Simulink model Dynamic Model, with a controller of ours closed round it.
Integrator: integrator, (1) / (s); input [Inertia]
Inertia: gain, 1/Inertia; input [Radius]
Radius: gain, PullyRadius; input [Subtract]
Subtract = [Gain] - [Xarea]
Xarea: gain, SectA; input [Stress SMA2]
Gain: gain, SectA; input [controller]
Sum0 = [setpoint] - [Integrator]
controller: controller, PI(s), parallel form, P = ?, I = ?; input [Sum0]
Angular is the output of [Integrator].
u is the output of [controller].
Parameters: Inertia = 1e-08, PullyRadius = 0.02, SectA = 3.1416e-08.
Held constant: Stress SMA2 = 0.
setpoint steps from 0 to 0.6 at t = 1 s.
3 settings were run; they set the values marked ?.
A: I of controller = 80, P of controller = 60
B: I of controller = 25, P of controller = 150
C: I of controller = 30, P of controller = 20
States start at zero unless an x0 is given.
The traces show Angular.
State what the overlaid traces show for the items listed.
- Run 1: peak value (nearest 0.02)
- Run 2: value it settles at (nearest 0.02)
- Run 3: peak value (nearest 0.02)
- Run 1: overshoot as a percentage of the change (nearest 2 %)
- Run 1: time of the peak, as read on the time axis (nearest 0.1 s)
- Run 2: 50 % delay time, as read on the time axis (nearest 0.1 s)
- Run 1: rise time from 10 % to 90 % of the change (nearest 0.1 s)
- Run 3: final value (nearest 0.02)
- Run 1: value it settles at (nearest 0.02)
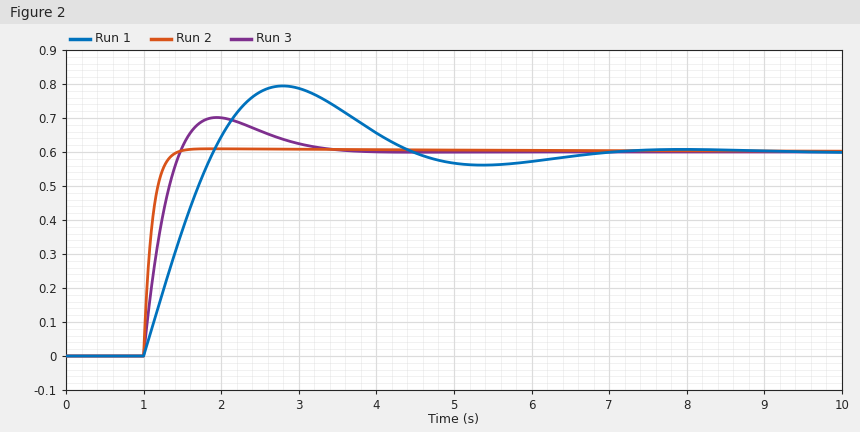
0.80
0.60
0.70
32 %
2.8 s
1.1 s
0.7 s
0.60
0.60
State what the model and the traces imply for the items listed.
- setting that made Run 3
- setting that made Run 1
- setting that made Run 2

A
C
B
